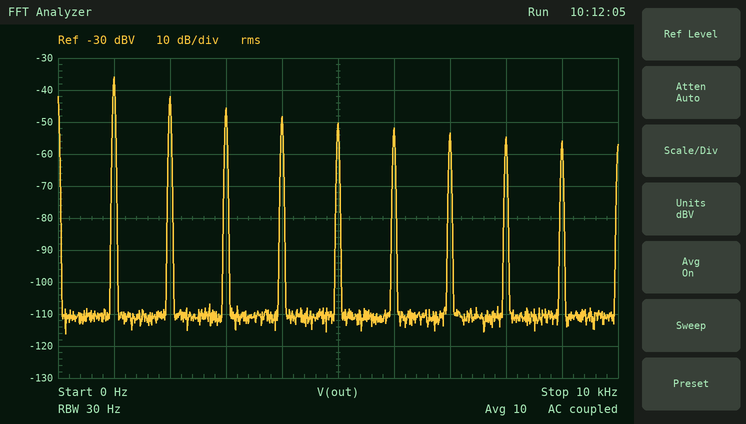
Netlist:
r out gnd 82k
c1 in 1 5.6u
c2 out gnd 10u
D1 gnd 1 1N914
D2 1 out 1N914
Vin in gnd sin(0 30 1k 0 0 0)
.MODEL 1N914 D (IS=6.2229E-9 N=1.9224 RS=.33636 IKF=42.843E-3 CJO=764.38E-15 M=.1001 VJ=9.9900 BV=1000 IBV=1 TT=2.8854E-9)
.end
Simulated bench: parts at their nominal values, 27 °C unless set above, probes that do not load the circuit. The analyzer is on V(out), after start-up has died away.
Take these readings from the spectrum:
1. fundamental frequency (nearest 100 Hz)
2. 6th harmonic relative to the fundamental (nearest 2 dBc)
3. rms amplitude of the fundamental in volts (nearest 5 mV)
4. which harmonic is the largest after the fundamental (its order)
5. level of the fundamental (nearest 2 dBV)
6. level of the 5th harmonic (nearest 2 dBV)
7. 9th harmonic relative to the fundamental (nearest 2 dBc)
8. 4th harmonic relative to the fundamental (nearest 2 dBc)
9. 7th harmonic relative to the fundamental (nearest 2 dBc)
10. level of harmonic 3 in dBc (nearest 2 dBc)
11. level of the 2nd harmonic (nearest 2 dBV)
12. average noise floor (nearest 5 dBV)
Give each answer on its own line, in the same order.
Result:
1.0 kHz
-16 dBc
15 mV
2
-36 dBV
-50 dBV
-20 dBc
-12 dBc
-18 dBc
-10 dBc
-42 dBV
-110 dBV
